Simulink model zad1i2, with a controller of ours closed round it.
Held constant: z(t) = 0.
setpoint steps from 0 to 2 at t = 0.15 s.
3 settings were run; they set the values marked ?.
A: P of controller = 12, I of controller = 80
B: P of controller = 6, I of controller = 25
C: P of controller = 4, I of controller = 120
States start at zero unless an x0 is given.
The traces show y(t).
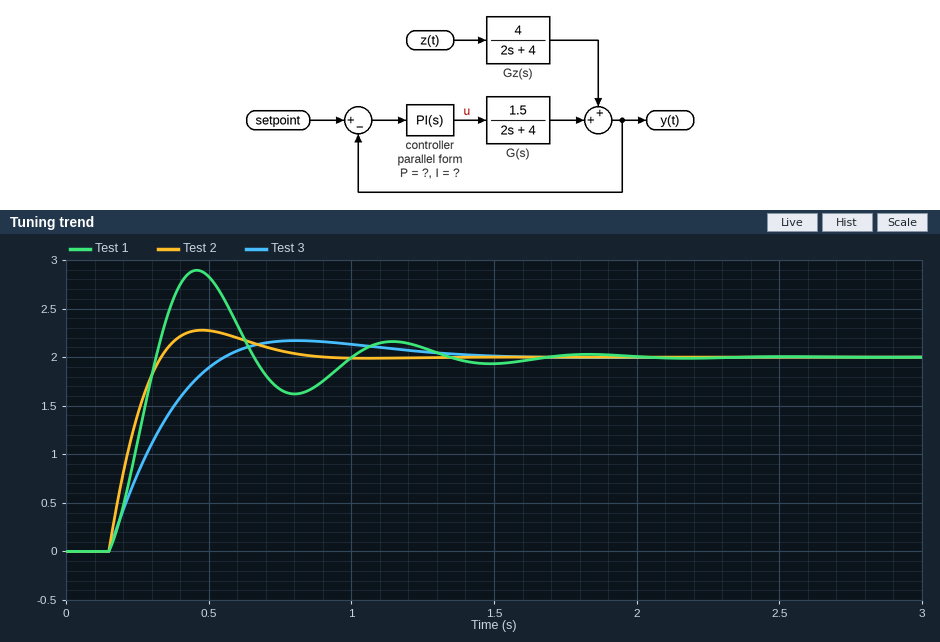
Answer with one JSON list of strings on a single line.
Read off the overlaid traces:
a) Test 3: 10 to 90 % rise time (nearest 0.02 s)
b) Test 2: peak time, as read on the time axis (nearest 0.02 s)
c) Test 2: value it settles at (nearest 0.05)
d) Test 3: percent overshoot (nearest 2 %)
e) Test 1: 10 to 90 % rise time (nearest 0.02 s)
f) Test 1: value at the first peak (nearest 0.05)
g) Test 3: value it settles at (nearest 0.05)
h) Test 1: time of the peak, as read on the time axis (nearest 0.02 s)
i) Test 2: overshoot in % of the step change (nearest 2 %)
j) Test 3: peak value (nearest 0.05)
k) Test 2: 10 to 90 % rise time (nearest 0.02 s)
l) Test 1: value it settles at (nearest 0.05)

["0.30 s", "0.48 s", "2.00", "8 %", "0.12 s", "2.90", "2.00", "0.46 s", "14 %", "2.15", "0.14 s", "2.00"]
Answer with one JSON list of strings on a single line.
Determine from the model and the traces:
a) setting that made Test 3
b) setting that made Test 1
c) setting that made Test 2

["B", "C", "A"]
